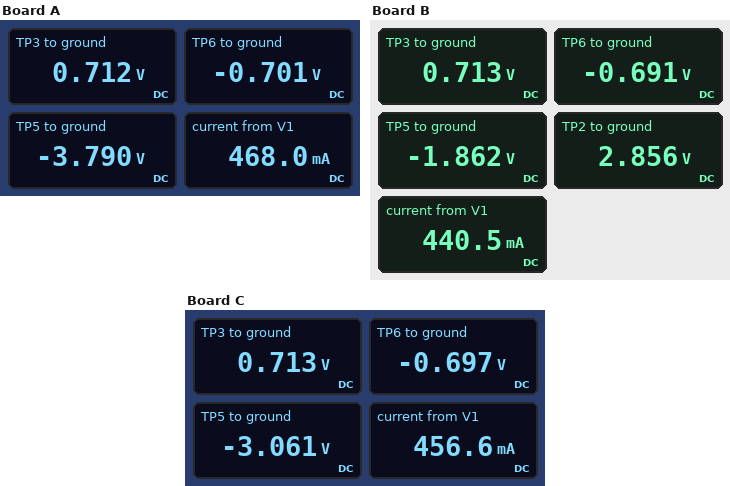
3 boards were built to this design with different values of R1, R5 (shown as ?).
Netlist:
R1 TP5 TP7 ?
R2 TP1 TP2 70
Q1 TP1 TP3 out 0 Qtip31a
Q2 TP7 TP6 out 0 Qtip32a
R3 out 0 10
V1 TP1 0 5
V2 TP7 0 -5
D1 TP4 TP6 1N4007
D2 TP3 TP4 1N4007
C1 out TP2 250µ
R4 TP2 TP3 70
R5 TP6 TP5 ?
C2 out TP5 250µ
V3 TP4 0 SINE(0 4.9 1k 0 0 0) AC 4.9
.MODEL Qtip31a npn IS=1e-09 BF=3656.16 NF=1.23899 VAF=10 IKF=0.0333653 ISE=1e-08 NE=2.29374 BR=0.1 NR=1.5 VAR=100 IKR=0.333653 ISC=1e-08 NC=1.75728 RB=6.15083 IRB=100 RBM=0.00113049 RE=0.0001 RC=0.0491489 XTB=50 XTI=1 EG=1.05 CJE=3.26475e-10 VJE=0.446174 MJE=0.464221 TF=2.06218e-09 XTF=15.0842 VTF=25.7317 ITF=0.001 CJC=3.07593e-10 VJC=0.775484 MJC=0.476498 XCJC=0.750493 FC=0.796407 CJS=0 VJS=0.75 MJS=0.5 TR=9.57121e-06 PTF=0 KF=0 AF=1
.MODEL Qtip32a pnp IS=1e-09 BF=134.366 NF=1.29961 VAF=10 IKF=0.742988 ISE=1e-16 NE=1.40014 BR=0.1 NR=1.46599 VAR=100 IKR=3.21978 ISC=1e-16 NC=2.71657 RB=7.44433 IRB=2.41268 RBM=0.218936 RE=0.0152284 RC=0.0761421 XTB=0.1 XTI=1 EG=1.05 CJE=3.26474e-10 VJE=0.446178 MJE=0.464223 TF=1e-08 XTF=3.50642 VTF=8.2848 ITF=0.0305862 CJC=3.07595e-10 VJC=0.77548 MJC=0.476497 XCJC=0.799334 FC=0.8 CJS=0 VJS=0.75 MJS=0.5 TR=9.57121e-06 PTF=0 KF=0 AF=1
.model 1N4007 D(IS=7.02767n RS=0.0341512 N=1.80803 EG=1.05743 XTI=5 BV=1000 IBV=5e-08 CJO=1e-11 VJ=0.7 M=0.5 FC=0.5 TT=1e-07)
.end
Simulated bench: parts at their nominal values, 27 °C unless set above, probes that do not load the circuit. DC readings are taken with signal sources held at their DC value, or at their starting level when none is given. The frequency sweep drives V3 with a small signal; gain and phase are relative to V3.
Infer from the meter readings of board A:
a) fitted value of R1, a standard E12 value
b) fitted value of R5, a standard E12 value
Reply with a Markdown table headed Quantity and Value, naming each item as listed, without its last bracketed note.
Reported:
| Quantity | Value |
|---|---|
| fitted value of R1, a standard E12 value | 47 Ω |
| fitted value of R5, a standard E12 value | 120 Ω |
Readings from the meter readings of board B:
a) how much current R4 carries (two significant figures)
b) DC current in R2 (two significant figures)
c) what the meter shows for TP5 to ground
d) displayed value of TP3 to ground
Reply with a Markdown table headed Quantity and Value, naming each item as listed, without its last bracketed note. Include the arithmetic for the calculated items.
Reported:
| Quantity | Value |
|---|---|
| how much current R4 carries | (2.856 V - 713 mV) / 70 Ω = 31 mA |
| DC current in R2 | (5 V - 2.856 V) / 70 Ω = 31 mA |
| what the meter shows for TP5 to ground | -1.862 V |
| displayed value of TP3 to ground | 0.713 V |
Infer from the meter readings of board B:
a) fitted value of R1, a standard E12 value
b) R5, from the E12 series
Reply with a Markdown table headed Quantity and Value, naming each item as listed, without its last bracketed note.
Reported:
| Quantity | Value |
|---|---|
| fitted value of R1, a standard E12 value | 150 Ω |
| R5, from the E12 series | 56 Ω |
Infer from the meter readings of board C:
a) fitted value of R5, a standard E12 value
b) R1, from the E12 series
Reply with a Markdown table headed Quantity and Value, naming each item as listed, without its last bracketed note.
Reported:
| Quantity | Value |
|---|---|
| fitted value of R5, a standard E12 value | 100 Ω |
| R1, from the E12 series | 82 Ω |
